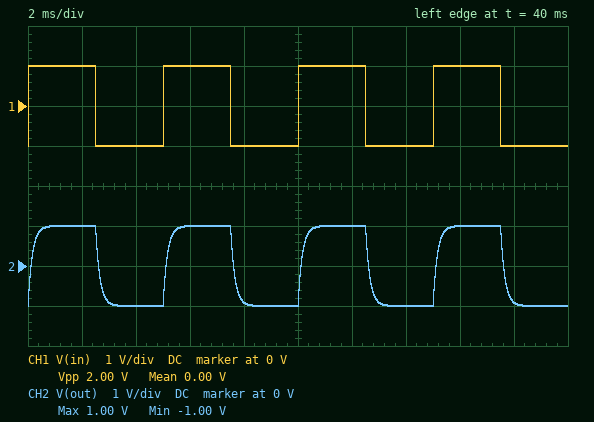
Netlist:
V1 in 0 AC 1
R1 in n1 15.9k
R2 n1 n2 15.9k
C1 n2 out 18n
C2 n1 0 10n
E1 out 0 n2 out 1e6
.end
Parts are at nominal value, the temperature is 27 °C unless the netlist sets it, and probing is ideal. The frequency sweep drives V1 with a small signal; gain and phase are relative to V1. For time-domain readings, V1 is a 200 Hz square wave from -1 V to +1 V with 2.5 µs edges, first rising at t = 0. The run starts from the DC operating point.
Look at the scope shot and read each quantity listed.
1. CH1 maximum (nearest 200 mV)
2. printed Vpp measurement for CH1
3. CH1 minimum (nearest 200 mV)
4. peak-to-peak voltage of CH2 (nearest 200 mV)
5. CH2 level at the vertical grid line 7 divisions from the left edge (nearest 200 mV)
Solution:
1.0 V
2.00 V
-1.0 V
2.0 V
-1.0 V
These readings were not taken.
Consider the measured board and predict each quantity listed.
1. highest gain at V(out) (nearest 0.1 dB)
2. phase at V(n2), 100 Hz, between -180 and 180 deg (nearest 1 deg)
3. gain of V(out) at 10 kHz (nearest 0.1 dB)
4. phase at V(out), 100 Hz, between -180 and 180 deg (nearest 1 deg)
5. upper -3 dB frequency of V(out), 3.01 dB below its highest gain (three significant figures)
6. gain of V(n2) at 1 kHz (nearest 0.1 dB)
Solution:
0 dB
-6 deg
-20.0 dB
-6 deg
1.00 kHz
-3.0 dB
